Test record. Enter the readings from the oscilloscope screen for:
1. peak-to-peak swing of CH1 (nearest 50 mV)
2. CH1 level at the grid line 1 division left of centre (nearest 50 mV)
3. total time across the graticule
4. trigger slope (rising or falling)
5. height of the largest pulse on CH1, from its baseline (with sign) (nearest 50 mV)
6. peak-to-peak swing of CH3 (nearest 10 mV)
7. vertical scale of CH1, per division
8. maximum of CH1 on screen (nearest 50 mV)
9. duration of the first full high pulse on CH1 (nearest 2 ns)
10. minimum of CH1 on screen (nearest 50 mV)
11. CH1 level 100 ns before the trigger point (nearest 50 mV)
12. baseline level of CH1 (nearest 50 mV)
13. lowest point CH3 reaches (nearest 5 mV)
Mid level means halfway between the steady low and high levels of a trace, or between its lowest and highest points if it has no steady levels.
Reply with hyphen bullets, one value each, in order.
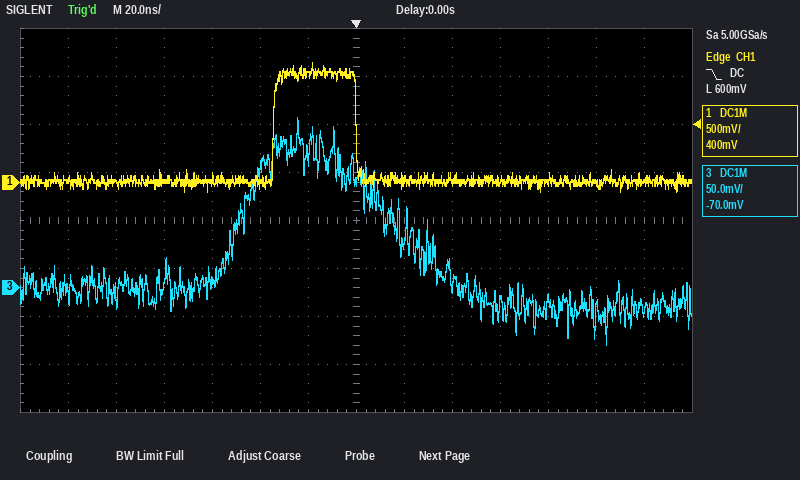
- 1.35 V
- 1.10 V
- 280 ns
- falling
- +1.25 V
- 240 mV
- 500 mV
- 1.25 V
- 34 ns
- -100 mV
- 0 mV
- 0 mV
- -60 mV
